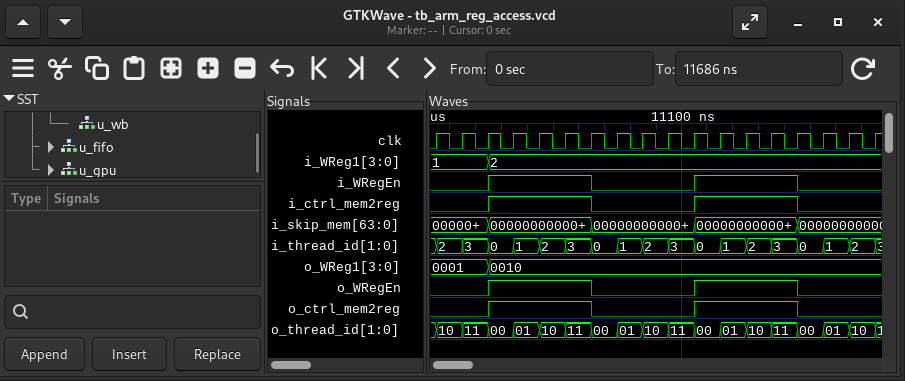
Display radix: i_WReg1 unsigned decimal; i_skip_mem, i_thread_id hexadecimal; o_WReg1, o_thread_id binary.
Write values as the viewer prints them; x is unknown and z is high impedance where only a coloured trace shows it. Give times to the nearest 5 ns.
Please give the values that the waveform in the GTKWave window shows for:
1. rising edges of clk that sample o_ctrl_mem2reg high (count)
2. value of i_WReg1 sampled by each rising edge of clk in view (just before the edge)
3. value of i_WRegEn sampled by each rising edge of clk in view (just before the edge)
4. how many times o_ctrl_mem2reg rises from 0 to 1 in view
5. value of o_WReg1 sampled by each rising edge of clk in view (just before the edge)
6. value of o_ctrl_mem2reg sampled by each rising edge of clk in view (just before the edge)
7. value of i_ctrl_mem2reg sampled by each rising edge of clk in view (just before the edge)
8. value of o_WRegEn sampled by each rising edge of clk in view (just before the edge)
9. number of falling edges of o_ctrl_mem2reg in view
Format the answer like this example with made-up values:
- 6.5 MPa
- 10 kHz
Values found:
- 8
- 1, 1, 1, 2, 2, 2, 2, 2, 2, 2, 2, 2, 2, 2, 2, 2, 2, 2
- 0 0 0 1 1 1 1 0 0 0 0 1 1 1 1 0 0 0
- 2
- 0001, 0001, 0001, 0010, 0010, 0010, 0010, 0010, 0010, 0010, 0010, 0010, 0010, 0010, 0010, 0010, 0010, 0010
- 0 0 0 1 1 1 1 0 0 0 0 1 1 1 1 0 0 0
- 0 0 0 1 1 1 1 0 0 0 0 1 1 1 1 0 0 0
- 0 0 0 1 1 1 1 0 0 0 0 1 1 1 1 0 0 0
- 2
